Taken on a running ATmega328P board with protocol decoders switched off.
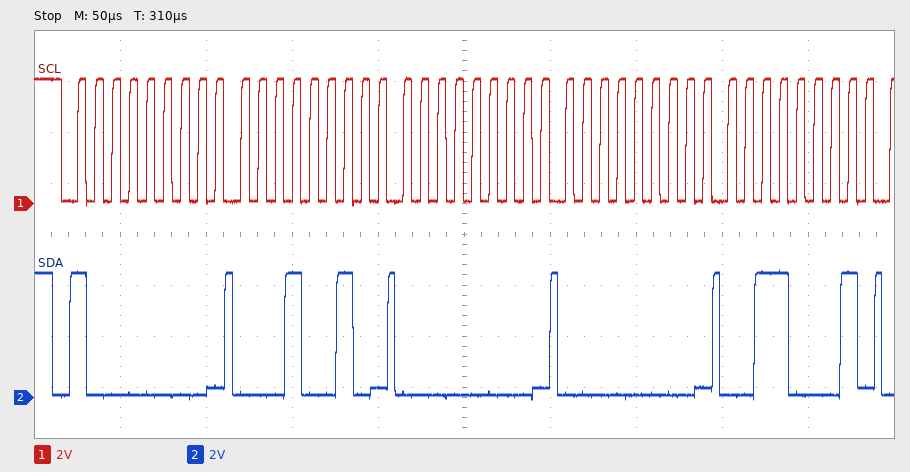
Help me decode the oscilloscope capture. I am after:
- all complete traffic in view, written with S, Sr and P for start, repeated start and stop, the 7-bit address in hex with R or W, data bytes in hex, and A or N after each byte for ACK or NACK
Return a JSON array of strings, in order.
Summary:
["S 40W A 12 A 00 A 00 A 31 A"]
